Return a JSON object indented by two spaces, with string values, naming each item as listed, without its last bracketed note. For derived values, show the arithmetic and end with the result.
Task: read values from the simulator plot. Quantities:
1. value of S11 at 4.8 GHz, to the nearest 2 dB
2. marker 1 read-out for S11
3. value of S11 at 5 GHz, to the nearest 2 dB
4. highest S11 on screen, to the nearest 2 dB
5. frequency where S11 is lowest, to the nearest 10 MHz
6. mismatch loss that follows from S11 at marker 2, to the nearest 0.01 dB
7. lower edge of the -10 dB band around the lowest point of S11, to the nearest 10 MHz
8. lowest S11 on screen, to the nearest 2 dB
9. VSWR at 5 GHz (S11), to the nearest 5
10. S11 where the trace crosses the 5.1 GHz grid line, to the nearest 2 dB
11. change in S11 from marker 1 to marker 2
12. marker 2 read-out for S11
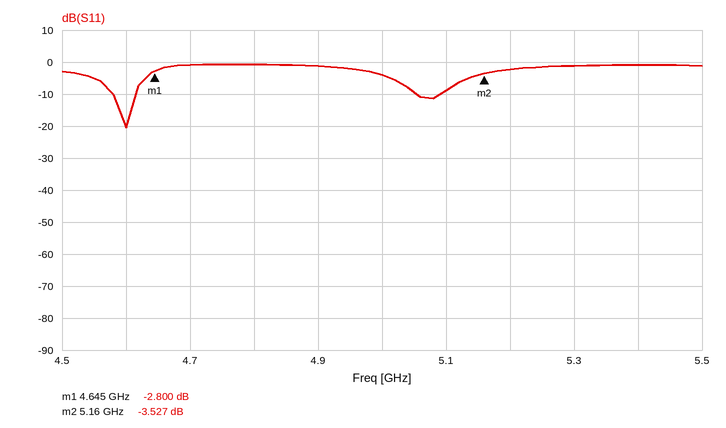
{
  "value of S11 at 4.8 GHz, to the nearest 2 dB": "0 dB",
  "marker 1 read-out for S11": "-2.800 dB",
  "value of S11 at 5 GHz, to the nearest 2 dB": "-4 dB",
  "highest S11 on screen, to the nearest 2 dB": "0 dB",
  "frequency where S11 is lowest, to the nearest 10 MHz": "4.60 GHz",
  "mismatch loss that follows from S11 at marker 2, to the nearest 0.01 dB": "−10 log10(1 − 10^(-3.527/10)) ≈ 2.55 dB",
  "lower edge of the -10 dB band around the lowest point of S11, to the nearest 10 MHz": "4.58 GHz",
  "lowest S11 on screen, to the nearest 2 dB": "-20 dB",
  "VSWR at 5 GHz (S11), to the nearest 5": "|Γ| = 10^(-4/20) = 0.6310; VSWR = (1 + 0.6310)/(1 − 0.6310) ≈ 4.42, so 5 to the nearest 5",
  "S11 where the trace crosses the 5.1 GHz grid line, to the nearest 2 dB": "-8 dB",
  "change in S11 from marker 1 to marker 2": "-3.527 − (-2.8) = -0.727 dB",
  "marker 2 read-out for S11": "-3.527 dB"
}
